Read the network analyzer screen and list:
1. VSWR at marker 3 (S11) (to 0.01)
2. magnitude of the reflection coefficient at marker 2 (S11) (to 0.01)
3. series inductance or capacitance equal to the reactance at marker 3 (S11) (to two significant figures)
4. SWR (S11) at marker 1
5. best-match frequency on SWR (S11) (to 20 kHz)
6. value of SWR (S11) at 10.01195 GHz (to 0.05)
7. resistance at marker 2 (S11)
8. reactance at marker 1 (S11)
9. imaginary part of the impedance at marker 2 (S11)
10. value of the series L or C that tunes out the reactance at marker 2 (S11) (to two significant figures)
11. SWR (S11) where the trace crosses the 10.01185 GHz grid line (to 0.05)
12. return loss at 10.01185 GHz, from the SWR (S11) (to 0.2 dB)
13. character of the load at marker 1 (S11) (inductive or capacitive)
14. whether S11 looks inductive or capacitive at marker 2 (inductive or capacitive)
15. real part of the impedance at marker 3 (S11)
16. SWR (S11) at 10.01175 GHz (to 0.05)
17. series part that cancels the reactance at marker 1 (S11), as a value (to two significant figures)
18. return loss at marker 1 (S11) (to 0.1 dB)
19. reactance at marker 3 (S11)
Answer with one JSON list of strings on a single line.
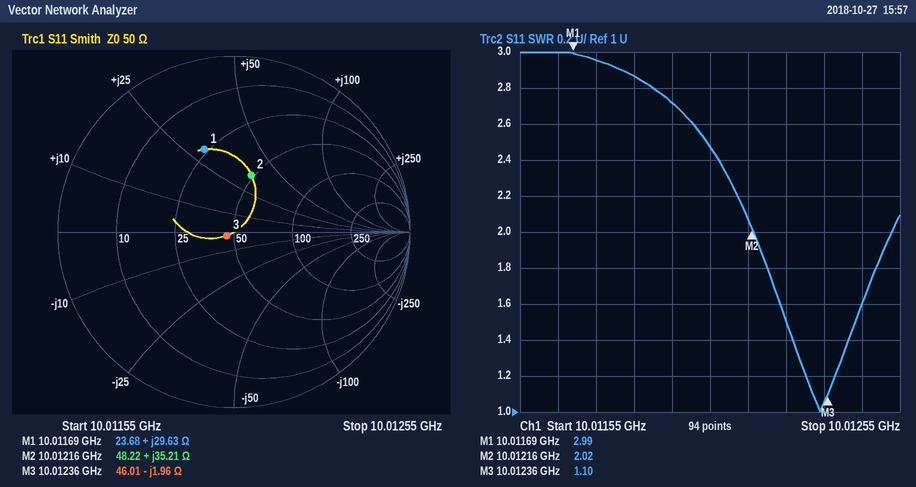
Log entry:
["1.10", "0.34", "8.1 pF", "2.99", "10.01234 GHz", "2.70", "48.22 Ω", "+29.63 Ω", "+35.21 Ω", "450 fF", "2.85", "6.4 dB", "inductive", "inductive", "46.01 Ω", "2.95", "540 fF", "6.0 dB", "-1.96 Ω"]
